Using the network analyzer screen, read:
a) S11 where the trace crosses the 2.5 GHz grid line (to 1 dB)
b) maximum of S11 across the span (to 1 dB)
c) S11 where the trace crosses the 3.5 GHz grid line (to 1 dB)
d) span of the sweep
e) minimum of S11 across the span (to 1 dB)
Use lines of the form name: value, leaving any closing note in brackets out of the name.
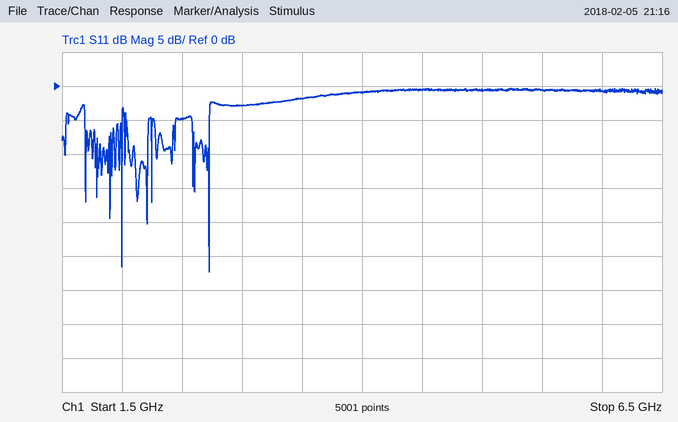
S11 where the trace crosses the 2.5 GHz grid line: -5 dB
maximum of S11 across the span: 0 dB
S11 where the trace crosses the 3.5 GHz grid line: -2 dB
span of the sweep: 5 GHz
minimum of S11 across the span: -27 dB
